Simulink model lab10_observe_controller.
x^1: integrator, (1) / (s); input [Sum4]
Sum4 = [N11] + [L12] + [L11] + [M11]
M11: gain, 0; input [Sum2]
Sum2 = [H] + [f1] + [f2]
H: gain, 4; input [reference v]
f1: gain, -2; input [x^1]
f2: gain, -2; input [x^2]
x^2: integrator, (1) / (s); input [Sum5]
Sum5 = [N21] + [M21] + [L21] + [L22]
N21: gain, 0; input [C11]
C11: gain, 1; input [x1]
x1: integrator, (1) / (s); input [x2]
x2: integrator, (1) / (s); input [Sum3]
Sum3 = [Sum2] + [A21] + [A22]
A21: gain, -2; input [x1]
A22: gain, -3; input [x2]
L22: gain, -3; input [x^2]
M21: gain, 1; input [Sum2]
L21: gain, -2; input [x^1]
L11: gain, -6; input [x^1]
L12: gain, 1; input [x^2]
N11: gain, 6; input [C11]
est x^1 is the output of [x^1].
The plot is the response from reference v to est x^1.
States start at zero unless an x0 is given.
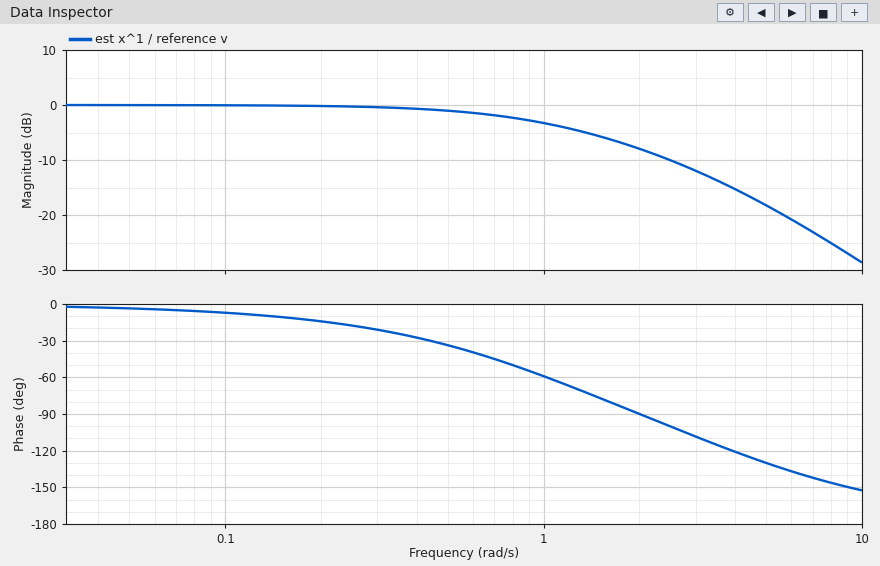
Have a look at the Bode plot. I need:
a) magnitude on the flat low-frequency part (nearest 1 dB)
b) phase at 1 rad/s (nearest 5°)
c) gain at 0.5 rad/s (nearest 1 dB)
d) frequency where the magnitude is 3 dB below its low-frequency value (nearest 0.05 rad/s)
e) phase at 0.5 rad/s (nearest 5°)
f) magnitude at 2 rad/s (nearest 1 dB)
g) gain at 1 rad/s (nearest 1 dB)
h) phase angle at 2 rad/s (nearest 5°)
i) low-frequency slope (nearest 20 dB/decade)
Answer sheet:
0 dB
-60°
-1 dB
0.95 rad/s
-35°
-8 dB
-3 dB
-90°
0 dB/decade
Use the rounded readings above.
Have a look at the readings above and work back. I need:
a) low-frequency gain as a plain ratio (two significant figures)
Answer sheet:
1.0
